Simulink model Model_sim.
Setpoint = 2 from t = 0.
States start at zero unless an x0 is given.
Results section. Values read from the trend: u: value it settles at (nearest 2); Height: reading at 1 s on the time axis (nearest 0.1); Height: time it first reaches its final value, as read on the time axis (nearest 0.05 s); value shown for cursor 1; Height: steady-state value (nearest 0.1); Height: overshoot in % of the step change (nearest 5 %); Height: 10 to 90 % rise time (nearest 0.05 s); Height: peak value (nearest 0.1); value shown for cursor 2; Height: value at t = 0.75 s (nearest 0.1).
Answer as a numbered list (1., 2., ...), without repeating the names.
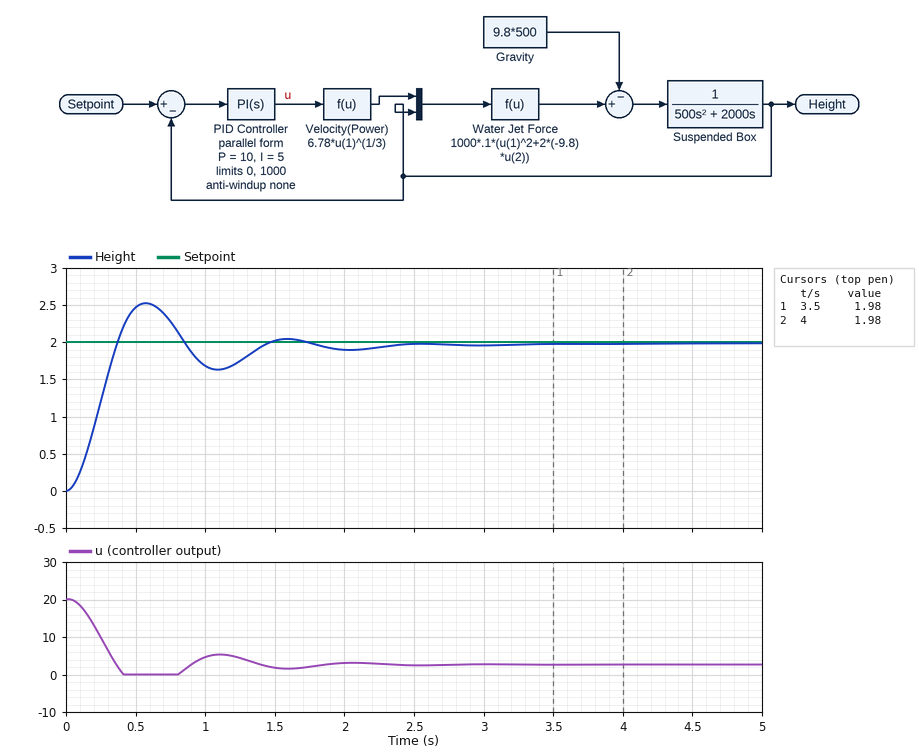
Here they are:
1. 2
2. 1.7
3. 0.35 s
4. 1.98
5. 2.0
6. 25 %
7. 0.25 s
8. 2.5
9. 1.98
10. 2.3
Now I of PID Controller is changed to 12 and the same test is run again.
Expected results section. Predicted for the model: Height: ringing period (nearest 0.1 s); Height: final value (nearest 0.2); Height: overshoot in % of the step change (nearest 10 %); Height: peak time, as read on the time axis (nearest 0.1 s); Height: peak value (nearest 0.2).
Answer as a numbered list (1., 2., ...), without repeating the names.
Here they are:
1. 1.1 s
2. 2.0
3. 40 %
4. 0.6 s
5. 2.8
